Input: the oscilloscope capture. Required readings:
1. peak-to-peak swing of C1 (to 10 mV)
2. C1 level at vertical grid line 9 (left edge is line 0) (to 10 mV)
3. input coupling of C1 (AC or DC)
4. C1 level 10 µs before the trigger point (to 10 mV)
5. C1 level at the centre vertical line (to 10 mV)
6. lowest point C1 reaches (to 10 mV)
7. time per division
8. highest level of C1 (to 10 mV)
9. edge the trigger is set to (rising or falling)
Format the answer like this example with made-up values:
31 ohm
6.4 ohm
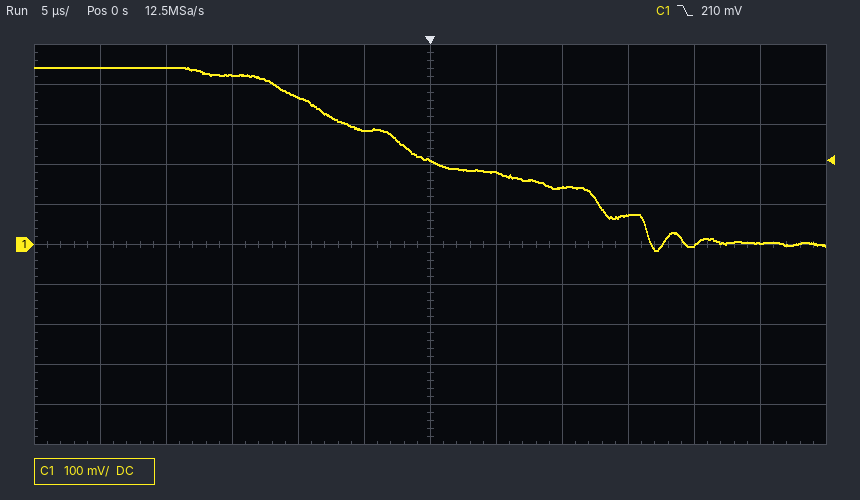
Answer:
460 mV
70 mV
DC
370 mV
210 mV
-20 mV
5 µs
440 mV
falling
